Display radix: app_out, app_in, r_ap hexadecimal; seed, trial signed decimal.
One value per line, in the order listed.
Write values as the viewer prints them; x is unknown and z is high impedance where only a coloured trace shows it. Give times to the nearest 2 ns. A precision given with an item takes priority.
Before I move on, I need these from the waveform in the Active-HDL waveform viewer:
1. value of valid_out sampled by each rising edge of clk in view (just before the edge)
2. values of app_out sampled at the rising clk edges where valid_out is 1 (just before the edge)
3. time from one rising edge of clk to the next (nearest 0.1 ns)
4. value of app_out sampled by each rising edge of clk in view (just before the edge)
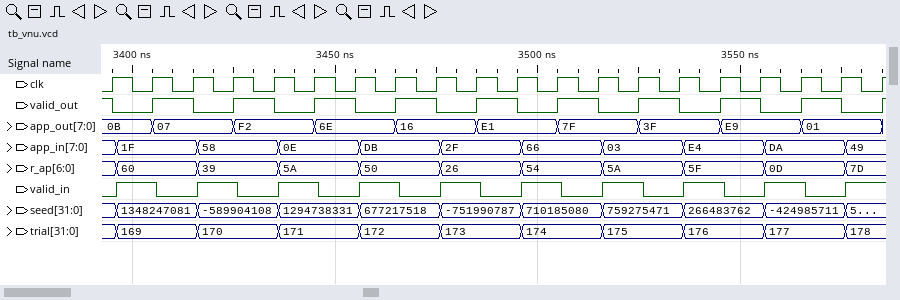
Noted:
1 0 1 0 1 0 1 0 1 0 1 0 1 0 1 0 1 0 1 0
0B, 07, F2, 6E, 16, E1, 7F, 3F, E9, 01
10 ns
0B, 0B, 07, 07, F2, F2, 6E, 6E, 16, 16, E1, E1, 7F, 7F, 3F, 3F, E9, E9, 01, 01
